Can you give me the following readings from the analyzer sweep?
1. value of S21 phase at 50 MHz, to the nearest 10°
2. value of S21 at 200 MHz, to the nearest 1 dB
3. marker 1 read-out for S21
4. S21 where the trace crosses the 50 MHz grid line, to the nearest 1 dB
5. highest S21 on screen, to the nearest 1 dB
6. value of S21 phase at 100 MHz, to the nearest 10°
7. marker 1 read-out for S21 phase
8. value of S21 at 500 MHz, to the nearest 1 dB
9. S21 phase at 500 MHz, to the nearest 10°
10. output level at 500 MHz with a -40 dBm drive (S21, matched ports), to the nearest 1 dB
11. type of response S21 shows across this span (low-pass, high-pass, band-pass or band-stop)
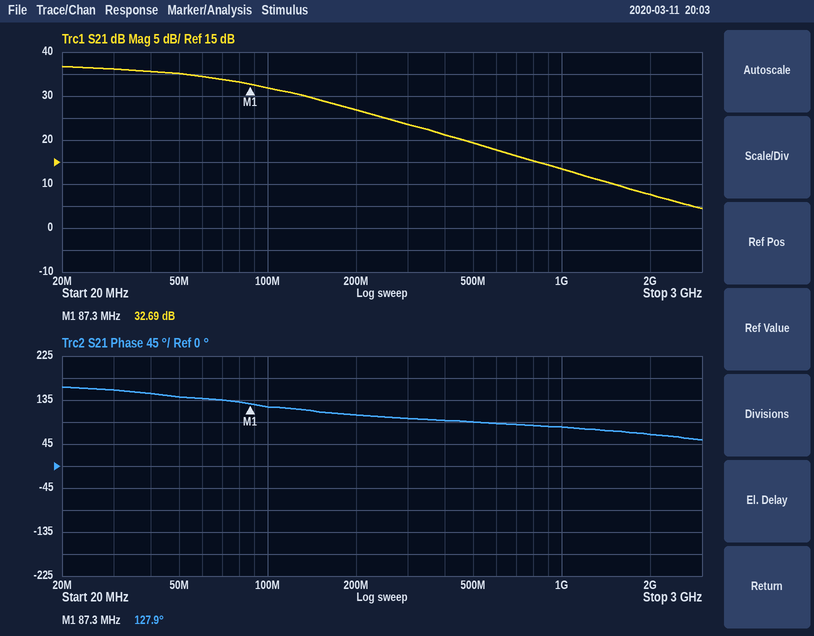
140°
27 dB
32.69 dB
35 dB
37 dB
120°
127.9°
19 dB
90°
-21 dBm
low-pass
